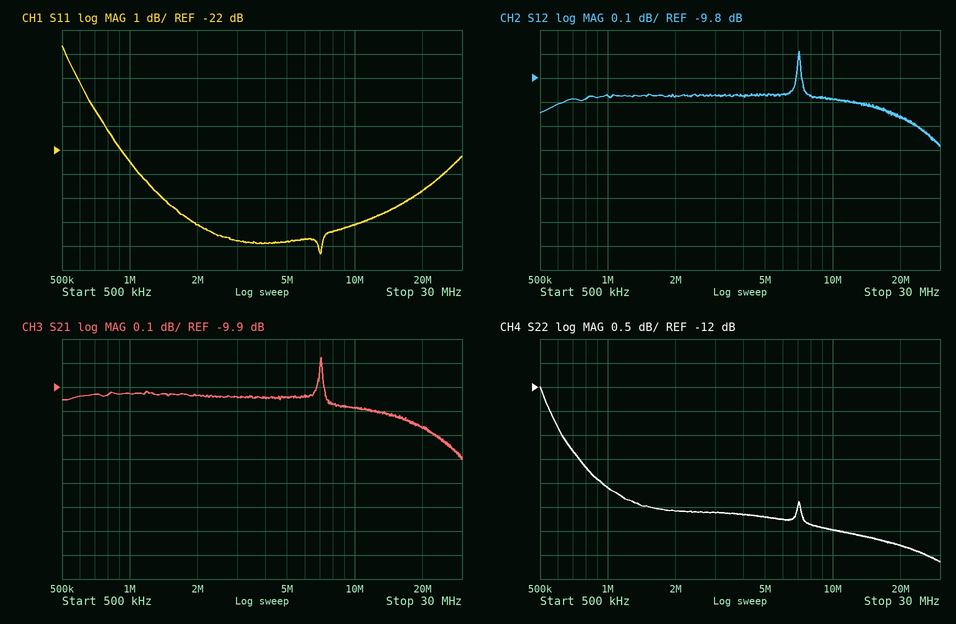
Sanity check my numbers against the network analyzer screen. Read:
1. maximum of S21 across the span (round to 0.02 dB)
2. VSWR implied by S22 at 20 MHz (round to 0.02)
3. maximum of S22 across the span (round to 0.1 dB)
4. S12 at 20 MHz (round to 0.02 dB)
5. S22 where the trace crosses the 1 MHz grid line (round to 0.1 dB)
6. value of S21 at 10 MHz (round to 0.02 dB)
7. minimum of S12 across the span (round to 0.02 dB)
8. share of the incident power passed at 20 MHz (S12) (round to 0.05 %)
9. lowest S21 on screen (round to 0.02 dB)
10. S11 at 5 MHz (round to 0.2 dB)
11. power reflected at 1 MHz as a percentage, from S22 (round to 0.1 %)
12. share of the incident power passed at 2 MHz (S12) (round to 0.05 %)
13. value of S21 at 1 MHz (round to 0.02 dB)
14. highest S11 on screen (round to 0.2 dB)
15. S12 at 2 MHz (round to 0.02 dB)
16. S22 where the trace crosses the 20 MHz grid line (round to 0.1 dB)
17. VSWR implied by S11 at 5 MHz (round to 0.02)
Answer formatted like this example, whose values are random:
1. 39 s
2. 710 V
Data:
1. -9.78 dB
2. 1.42
3. -12.0 dB
4. -9.96 dB
5. -14.1 dB
6. -9.98 dB
7. -10.08 dB
8. 10.10 %
9. -10.20 dB
10. -25.8 dB
11. 3.9 %
12. 10.30 %
13. -9.92 dB
14. -17.6 dB
15. -9.88 dB
16. -15.3 dB
17. 1.10
